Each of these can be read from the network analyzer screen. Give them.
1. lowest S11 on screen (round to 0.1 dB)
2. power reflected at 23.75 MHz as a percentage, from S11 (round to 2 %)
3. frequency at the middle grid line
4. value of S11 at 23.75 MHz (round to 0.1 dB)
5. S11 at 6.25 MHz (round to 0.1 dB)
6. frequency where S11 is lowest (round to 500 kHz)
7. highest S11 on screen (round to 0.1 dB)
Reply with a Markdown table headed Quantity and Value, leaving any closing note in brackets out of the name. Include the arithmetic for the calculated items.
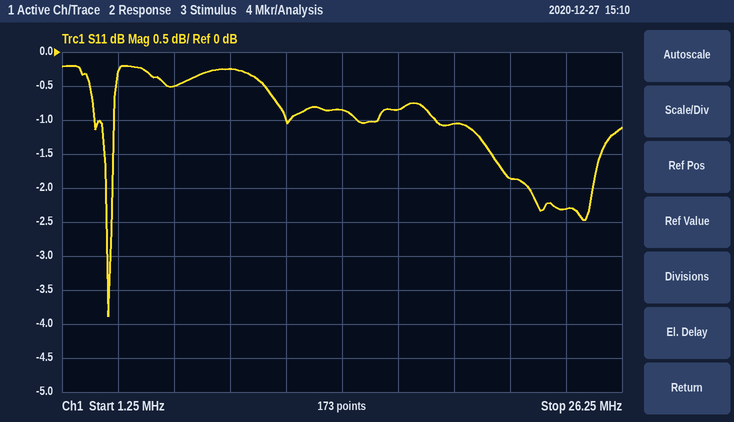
| Quantity | Value |
|---|---|
| lowest S11 on screen | -3.9 dB |
| power reflected at 23.75 MHz as a percentage, from S11 | 10^(-2.3/10) ≈ 58.9 %, so 58 % to the nearest 2 % |
| frequency at the middle grid line | 13.75 MHz |
| value of S11 at 23.75 MHz | -2.3 dB |
| S11 at 6.25 MHz | -0.5 dB |
| frequency where S11 is lowest | 3.5 MHz |
| highest S11 on screen | -0.2 dB |
